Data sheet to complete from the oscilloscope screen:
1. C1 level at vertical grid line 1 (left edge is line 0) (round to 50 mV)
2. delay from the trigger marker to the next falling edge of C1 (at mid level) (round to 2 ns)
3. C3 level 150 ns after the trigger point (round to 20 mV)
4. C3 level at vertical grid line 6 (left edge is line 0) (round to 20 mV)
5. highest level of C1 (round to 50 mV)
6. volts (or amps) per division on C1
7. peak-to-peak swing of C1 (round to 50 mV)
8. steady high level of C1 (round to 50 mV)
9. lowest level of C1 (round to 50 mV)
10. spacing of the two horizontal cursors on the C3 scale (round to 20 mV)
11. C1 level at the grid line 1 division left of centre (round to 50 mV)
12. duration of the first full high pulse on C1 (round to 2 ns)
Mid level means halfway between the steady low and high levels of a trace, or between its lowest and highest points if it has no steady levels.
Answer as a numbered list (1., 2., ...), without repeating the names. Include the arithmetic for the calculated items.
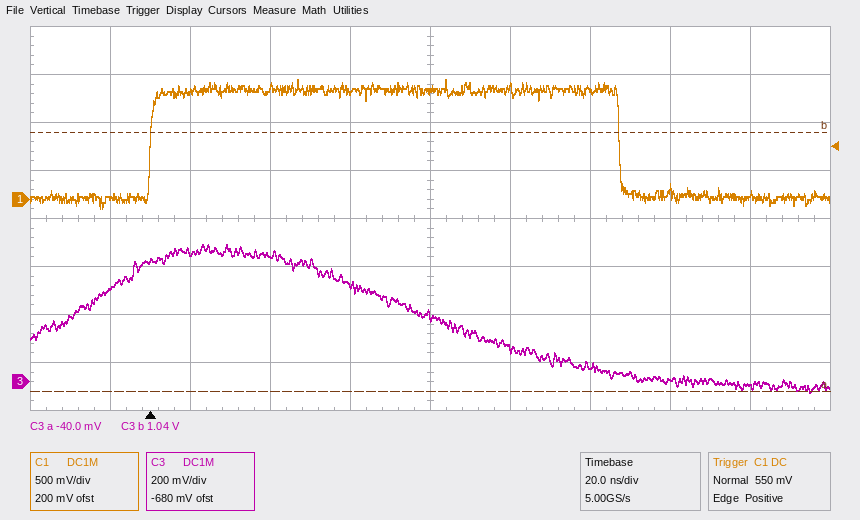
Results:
1. 50 mV
2. 118 ns
3. -20 mV
4. 140 mV
5. 1.25 V
6. 500 mV
7. 1.25 V − (-100 mV) = 1.35 V
8. 1.15 V
9. -100 mV
10. 1.08 V
11. 1.15 V
12. 118 ns
